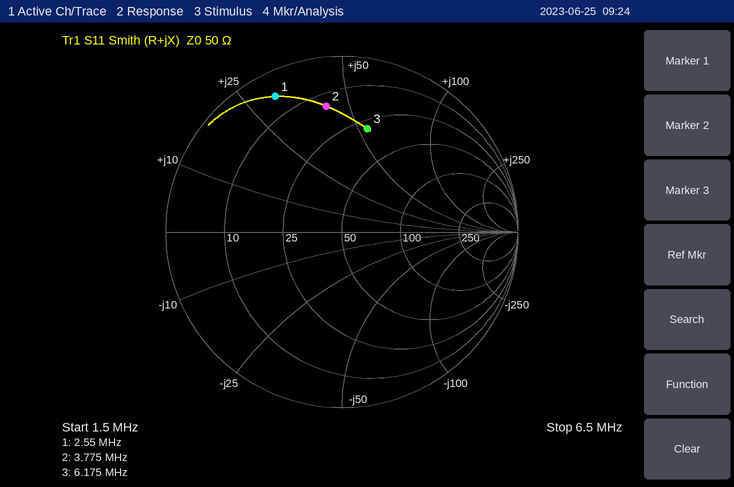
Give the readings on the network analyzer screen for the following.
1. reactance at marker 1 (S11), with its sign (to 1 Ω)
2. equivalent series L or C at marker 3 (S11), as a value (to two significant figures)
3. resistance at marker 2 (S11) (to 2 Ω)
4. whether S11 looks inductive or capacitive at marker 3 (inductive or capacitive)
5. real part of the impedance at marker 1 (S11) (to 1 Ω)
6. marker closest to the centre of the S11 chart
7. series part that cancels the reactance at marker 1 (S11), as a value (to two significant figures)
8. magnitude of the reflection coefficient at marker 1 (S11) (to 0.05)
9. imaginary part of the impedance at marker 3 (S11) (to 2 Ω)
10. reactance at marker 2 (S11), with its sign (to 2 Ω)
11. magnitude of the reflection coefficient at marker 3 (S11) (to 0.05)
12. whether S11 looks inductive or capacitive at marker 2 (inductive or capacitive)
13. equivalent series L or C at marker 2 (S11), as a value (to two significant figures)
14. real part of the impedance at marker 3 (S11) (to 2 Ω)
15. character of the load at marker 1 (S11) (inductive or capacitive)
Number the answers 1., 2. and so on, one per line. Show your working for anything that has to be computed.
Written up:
1. +31 Ω
2. L = 54 Ω/(2π × 6.175 MHz) ≈ 1.4 µH
3. 14 Ω
4. inductive
5. 5 Ω
6. marker 3
7. C = 1/(2π × 2.55 MHz × 31 Ω) ≈ 2.0 nF
8. 0.85
9. +54 Ω
10. +42 Ω
11. 0.60
12. inductive
13. L = 42 Ω/(2π × 3.775 MHz) ≈ 1.8 µH
14. 30 Ω
15. inductive
